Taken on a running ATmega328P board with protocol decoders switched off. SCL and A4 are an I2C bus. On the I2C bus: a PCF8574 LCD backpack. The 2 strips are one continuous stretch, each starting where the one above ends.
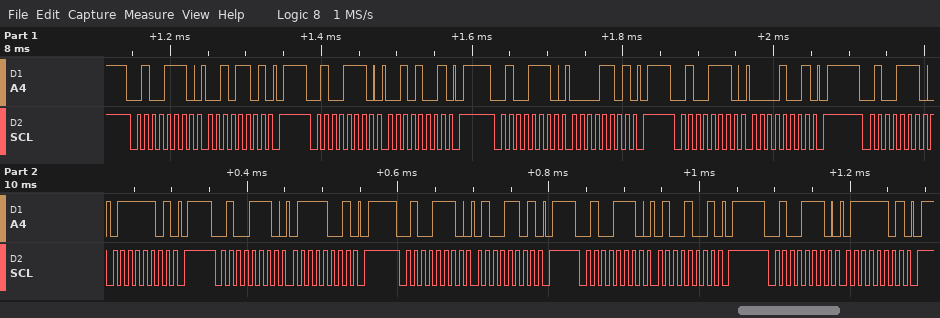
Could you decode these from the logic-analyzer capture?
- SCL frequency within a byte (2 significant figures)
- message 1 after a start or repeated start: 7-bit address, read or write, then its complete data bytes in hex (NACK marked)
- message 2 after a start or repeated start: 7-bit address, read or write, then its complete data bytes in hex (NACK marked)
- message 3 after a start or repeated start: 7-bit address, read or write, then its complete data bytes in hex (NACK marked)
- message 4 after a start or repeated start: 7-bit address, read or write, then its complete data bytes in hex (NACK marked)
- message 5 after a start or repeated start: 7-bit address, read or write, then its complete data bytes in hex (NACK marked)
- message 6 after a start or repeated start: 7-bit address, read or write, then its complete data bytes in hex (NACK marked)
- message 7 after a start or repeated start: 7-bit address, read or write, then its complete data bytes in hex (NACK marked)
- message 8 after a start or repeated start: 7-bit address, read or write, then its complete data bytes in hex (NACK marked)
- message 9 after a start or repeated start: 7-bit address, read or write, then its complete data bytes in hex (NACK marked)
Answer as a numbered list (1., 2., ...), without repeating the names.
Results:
1. 100 kHz
2. 0x27 write: 2D
3. 0x27 write: 29
4. 0x27 write: 0D
5. 0x27 write: 09
6. 0x27 write: 7D
7. 0x27 write: 79
8. 0x27 write: 4D
9. 0x27 write: 49
10. 0x27 write: 7D
